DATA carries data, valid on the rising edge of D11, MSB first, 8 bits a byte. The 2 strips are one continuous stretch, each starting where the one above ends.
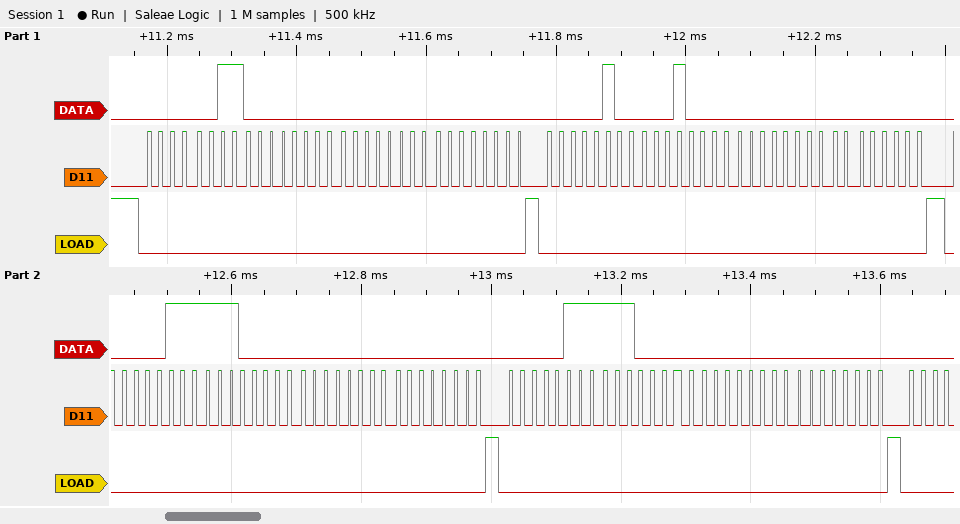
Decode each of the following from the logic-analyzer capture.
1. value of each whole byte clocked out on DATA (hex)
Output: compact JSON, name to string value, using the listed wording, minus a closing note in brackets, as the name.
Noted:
{"value of each whole byte clocked out on DATA": "0x03 0x00 0x00 0x00 0x04 0x10 0x00 0x00 0x07 0xE0 0x00 0x00 0x07 0xE0 0x00 0x00"}
